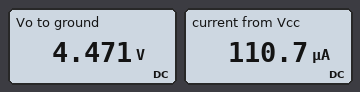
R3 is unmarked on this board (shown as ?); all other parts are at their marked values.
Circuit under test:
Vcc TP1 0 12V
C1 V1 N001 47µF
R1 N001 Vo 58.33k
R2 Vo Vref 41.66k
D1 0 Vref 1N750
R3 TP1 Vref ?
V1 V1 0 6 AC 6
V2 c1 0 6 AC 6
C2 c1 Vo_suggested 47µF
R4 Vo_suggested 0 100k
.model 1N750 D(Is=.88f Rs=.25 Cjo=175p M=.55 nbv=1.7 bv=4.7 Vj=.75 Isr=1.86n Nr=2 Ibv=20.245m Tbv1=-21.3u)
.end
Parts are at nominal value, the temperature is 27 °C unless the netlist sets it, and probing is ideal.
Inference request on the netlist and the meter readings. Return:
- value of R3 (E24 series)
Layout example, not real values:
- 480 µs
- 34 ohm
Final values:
- 68 kΩ
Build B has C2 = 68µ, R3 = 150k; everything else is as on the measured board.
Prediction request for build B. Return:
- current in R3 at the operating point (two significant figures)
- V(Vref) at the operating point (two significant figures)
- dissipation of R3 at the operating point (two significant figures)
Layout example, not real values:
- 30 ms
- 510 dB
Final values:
- 50 µA
- 4.4 V
- 380 µW
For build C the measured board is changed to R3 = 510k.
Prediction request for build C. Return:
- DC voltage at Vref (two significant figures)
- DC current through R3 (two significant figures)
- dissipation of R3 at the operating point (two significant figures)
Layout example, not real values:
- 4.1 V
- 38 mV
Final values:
- 4.4 V
- 15 µA
- 110 µW
